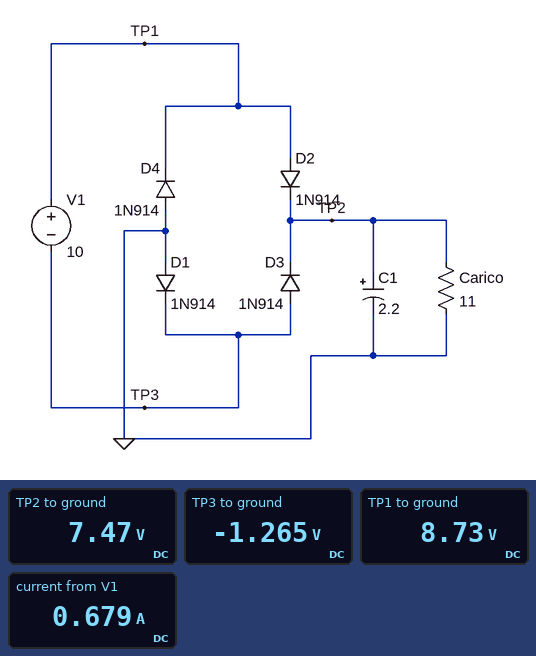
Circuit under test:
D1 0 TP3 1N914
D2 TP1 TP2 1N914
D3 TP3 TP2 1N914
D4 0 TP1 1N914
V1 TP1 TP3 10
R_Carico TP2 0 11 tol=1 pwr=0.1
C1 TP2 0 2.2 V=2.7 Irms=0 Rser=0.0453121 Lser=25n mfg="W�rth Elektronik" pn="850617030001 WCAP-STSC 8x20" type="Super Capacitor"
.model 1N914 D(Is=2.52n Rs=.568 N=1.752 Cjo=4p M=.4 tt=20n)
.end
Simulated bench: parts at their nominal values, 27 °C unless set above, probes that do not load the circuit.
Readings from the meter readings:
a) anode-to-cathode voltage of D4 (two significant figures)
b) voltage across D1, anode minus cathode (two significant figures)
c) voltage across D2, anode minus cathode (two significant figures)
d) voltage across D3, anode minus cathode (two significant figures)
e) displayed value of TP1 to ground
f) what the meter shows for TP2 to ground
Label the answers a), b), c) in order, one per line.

a) -8.7 V
b) 1.3 V
c) 1.3 V
d) -8.7 V
e) 8.73 V
f) 7.47 V
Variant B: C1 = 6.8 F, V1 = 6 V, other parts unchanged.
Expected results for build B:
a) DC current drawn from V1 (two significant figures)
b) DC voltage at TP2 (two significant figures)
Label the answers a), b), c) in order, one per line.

a) 350 mA
b) 3.9 V
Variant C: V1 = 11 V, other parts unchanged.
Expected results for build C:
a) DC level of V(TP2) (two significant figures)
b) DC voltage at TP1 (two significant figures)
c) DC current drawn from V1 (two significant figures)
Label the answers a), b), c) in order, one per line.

a) 8.4 V
b) 9.7 V
c) 760 mA
